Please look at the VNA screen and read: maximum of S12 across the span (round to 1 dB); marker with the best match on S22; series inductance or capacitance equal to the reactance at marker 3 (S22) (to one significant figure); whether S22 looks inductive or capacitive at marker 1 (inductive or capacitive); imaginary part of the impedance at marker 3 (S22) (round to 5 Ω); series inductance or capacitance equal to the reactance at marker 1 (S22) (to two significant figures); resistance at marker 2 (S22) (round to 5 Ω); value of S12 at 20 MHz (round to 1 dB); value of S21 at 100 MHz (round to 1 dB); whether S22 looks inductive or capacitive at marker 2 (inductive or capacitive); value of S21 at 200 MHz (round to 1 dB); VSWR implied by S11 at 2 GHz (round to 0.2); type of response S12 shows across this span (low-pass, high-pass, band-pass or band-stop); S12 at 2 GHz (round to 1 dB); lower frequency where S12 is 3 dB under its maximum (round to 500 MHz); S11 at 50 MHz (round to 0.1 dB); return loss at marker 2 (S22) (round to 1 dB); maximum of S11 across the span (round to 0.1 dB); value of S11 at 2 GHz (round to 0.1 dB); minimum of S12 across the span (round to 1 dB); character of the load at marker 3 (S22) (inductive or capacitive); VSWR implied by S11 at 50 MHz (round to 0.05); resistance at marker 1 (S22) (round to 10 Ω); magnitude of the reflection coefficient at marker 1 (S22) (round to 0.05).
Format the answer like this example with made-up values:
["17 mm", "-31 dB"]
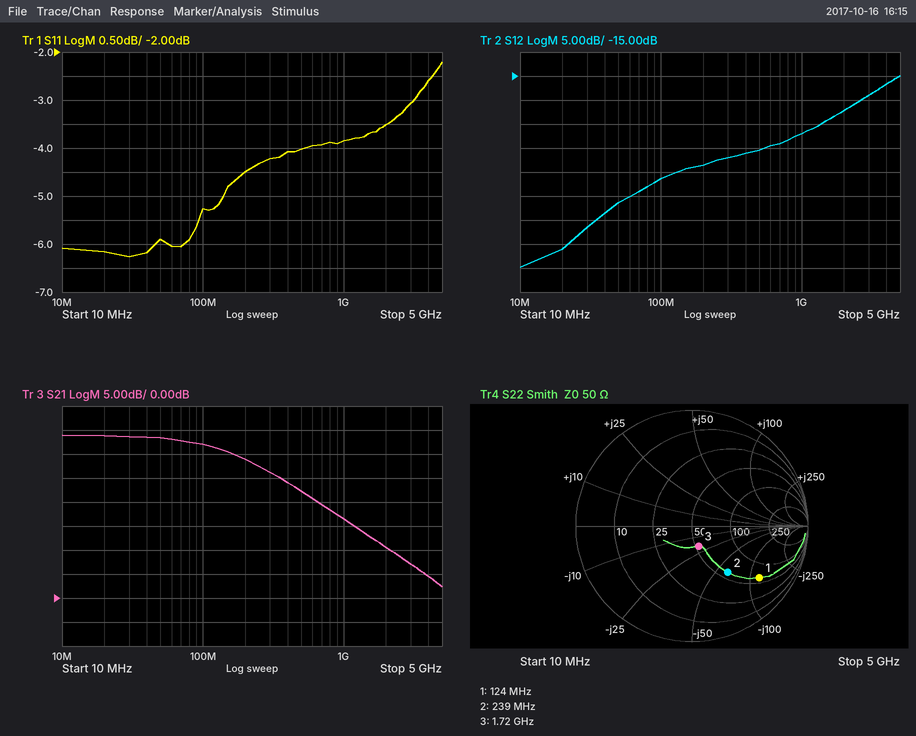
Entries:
["-15 dB", "marker 3", "5 pF", "capacitive", "-20 Ω", "11 pF", "60 Ω", "-51 dB", "32 dB", "capacitive", "29 dB", "5.0", "high-pass", "-22 dB", "3.5 GHz", "-5.9 dB", "6 dB", "-2.2 dB", "-3.5 dB", "-55 dB", "capacitive", "3.05", "60 Ω", "0.75"]
